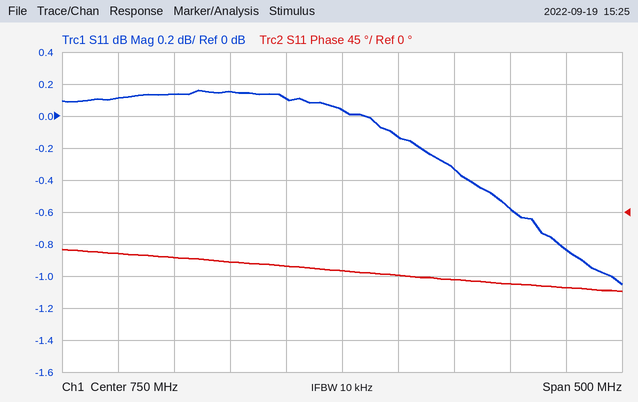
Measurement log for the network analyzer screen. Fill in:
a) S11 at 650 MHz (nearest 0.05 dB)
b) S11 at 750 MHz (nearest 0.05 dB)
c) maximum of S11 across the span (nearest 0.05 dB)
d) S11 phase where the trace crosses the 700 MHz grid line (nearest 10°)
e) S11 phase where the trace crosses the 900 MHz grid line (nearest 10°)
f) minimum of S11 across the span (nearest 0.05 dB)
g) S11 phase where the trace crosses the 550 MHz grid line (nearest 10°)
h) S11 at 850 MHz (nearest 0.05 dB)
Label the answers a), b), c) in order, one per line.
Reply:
a) 0.15 dB
b) 0.05 dB
c) 0.15 dB
d) -80°
e) -100°
f) -1.05 dB
g) -60°
h) -0.35 dB
